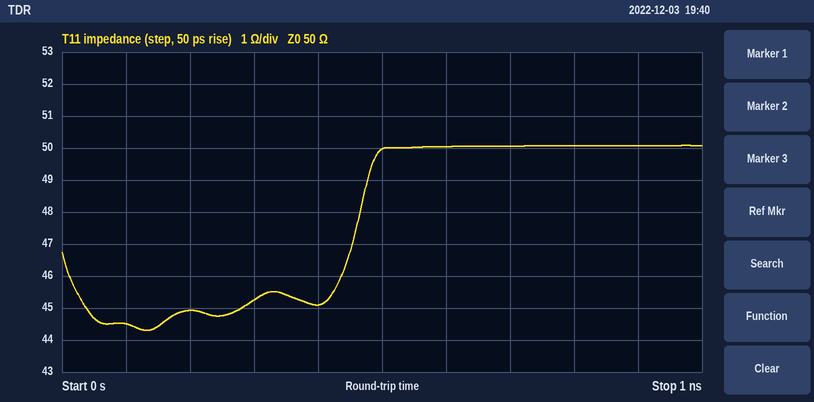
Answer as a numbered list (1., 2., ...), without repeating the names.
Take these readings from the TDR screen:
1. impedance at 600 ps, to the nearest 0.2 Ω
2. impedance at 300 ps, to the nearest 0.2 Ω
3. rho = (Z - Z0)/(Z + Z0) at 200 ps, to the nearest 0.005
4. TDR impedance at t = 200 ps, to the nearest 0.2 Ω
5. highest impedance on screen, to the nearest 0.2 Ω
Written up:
1. 50.0 Ω
2. 45.2 Ω
3. -0.055
4. 45.0 Ω
5. 50.0 Ω
